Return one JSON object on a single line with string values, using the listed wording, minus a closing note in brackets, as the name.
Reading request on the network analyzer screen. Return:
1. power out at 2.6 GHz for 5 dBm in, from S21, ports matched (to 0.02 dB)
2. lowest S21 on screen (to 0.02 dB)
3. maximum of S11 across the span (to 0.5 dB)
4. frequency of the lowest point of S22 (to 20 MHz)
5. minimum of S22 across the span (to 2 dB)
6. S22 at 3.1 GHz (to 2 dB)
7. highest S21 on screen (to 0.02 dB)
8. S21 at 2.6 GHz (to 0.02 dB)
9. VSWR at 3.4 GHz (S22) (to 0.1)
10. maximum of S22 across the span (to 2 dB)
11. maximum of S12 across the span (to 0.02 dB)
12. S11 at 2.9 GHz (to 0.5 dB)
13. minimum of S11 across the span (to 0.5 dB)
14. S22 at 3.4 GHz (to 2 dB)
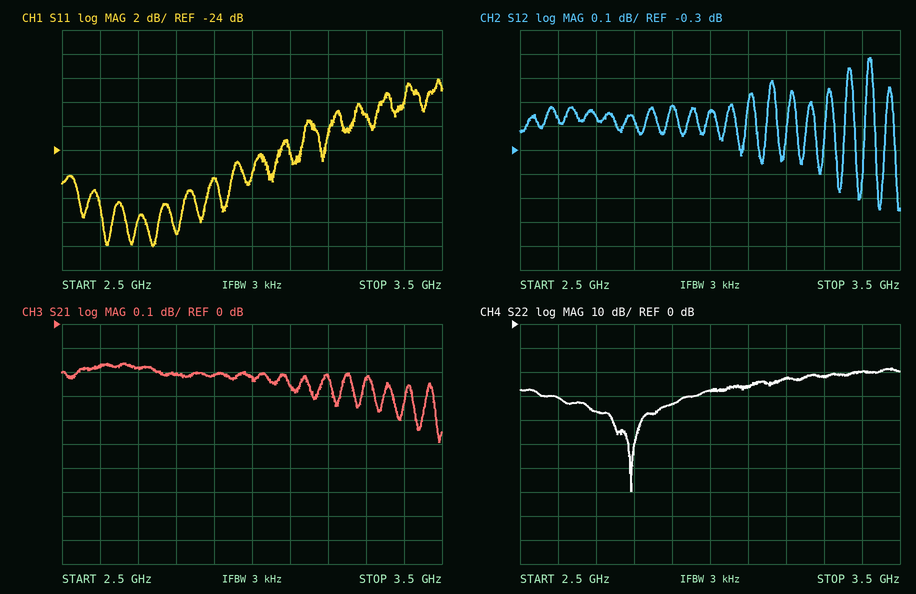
{"power out at 2.6 GHz for 5 dBm in, from S21, ports matched": "4.82 dBm", "lowest S21 on screen": "-0.50 dB", "maximum of S11 across the span": "-18.0 dB", "frequency of the lowest point of S22": "2.80 GHz", "minimum of S22 across the span": "-70 dB", "S22 at 3.1 GHz": "-26 dB", "highest S21 on screen": "-0.16 dB", "S21 at 2.6 GHz": "-0.18 dB", "VSWR at 3.4 GHz (S22)": "1.2", "maximum of S22 across the span": "-18 dB", "maximum of S12 across the span": "0.08 dB", "S11 at 2.9 GHz": "-26.5 dB", "minimum of S11 across the span": "-32.0 dB", "S22 at 3.4 GHz": "-20 dB"}
